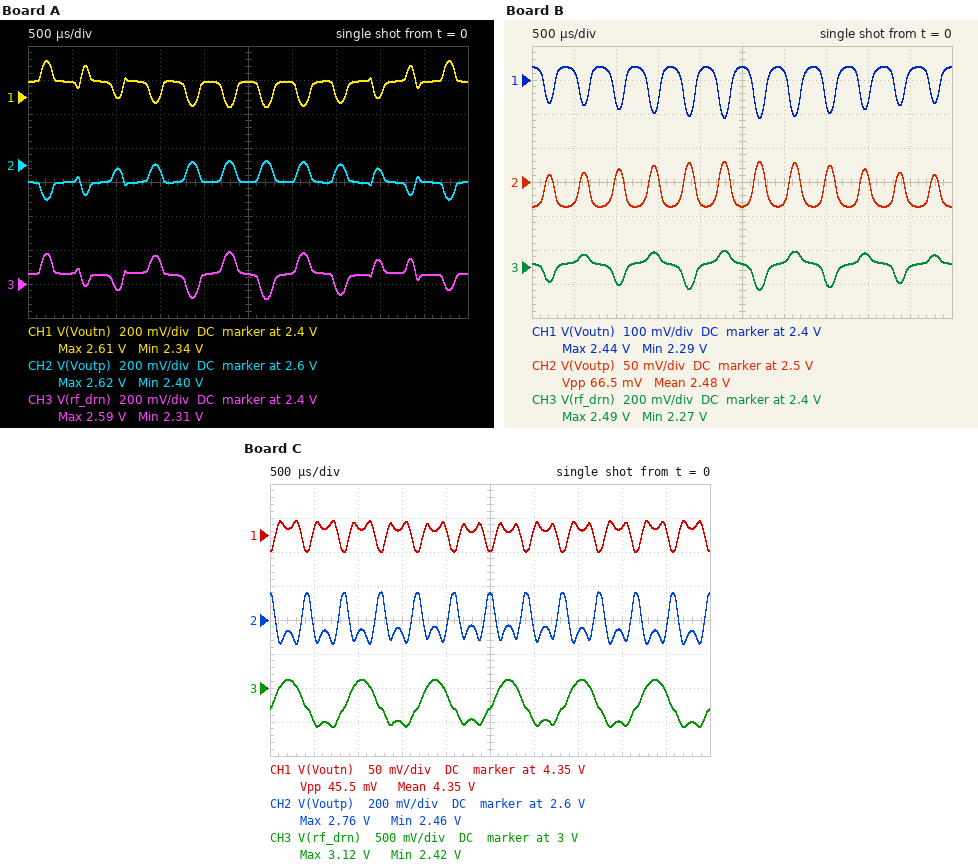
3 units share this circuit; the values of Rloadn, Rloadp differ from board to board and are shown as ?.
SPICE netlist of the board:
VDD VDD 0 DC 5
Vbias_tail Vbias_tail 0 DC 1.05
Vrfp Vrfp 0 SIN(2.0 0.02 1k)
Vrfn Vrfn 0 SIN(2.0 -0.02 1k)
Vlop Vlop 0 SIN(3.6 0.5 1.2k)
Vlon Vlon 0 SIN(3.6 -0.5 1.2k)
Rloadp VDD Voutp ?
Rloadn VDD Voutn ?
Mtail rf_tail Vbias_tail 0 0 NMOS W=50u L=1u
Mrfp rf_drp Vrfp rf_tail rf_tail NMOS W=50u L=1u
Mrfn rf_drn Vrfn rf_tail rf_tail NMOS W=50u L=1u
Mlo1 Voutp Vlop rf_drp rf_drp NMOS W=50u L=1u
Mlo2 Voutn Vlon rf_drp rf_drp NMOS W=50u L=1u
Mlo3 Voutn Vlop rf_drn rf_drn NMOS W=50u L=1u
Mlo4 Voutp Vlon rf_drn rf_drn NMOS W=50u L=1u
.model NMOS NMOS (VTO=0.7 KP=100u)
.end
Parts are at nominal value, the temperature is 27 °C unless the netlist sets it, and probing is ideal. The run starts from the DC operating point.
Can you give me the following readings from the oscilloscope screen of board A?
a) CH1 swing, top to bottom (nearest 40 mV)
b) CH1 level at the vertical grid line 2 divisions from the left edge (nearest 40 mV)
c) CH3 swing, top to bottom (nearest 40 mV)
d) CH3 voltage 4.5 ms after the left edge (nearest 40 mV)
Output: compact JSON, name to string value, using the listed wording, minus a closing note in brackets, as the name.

{"CH1 swing, top to bottom": "280 mV", "CH1 level at the vertical grid line 2 divisions from the left edge": "2.40 V", "CH3 swing, top to bottom": "280 mV", "CH3 voltage 4.5 ms after the left edge": "2.44 V"}
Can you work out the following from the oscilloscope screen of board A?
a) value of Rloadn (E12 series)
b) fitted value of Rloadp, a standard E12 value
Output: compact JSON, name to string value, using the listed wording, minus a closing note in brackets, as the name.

{"value of Rloadn": "18 kΩ", "fitted value of Rloadp, a standard E12 value": "15 kΩ"}
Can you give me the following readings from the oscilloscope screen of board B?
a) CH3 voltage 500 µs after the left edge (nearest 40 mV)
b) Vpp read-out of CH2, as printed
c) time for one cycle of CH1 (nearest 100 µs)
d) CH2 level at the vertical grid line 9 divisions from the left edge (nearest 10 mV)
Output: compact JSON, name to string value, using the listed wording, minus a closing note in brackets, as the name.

{"CH3 voltage 500 µs after the left edge": "2.44 V", "Vpp read-out of CH2, as printed": "66.5 mV", "time for one cycle of CH1": "400 µs", "CH2 level at the vertical grid line 9 divisions from the left edge": "2.47 V"}
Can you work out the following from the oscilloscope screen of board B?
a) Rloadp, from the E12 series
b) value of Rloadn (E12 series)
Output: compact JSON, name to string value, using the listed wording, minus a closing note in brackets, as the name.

{"Rloadp, from the E12 series": "12 kΩ", "value of Rloadn": "27 kΩ"}
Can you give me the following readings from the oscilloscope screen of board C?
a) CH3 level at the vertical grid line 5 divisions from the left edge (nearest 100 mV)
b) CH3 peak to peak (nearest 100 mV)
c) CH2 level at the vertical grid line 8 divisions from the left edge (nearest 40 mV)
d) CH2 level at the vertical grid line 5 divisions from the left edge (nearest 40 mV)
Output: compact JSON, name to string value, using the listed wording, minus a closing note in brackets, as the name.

{"CH3 level at the vertical grid line 5 divisions from the left edge": "2.7 V", "CH3 peak to peak": "700 mV", "CH2 level at the vertical grid line 8 divisions from the left edge": "2.52 V", "CH2 level at the vertical grid line 5 divisions from the left edge": "2.76 V"}
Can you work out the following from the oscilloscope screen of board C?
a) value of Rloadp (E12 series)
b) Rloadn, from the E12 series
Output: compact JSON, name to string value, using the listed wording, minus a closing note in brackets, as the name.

{"value of Rloadp": "22 kΩ", "Rloadn, from the E12 series": "3.3 kΩ"}
